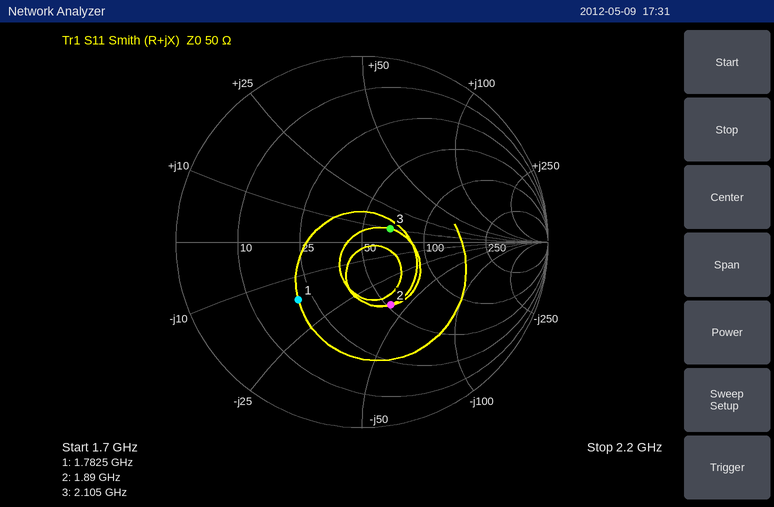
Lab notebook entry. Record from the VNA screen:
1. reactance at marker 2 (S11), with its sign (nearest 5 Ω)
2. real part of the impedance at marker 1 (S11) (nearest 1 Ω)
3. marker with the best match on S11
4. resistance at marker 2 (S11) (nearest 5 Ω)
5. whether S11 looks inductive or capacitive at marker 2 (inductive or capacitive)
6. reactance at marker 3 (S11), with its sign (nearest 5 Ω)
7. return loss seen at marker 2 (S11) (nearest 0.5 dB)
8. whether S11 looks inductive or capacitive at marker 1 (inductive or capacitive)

-40 Ω
21 Ω
marker 3
50 Ω
capacitive
+10 Ω
8.5 dB
capacitive
